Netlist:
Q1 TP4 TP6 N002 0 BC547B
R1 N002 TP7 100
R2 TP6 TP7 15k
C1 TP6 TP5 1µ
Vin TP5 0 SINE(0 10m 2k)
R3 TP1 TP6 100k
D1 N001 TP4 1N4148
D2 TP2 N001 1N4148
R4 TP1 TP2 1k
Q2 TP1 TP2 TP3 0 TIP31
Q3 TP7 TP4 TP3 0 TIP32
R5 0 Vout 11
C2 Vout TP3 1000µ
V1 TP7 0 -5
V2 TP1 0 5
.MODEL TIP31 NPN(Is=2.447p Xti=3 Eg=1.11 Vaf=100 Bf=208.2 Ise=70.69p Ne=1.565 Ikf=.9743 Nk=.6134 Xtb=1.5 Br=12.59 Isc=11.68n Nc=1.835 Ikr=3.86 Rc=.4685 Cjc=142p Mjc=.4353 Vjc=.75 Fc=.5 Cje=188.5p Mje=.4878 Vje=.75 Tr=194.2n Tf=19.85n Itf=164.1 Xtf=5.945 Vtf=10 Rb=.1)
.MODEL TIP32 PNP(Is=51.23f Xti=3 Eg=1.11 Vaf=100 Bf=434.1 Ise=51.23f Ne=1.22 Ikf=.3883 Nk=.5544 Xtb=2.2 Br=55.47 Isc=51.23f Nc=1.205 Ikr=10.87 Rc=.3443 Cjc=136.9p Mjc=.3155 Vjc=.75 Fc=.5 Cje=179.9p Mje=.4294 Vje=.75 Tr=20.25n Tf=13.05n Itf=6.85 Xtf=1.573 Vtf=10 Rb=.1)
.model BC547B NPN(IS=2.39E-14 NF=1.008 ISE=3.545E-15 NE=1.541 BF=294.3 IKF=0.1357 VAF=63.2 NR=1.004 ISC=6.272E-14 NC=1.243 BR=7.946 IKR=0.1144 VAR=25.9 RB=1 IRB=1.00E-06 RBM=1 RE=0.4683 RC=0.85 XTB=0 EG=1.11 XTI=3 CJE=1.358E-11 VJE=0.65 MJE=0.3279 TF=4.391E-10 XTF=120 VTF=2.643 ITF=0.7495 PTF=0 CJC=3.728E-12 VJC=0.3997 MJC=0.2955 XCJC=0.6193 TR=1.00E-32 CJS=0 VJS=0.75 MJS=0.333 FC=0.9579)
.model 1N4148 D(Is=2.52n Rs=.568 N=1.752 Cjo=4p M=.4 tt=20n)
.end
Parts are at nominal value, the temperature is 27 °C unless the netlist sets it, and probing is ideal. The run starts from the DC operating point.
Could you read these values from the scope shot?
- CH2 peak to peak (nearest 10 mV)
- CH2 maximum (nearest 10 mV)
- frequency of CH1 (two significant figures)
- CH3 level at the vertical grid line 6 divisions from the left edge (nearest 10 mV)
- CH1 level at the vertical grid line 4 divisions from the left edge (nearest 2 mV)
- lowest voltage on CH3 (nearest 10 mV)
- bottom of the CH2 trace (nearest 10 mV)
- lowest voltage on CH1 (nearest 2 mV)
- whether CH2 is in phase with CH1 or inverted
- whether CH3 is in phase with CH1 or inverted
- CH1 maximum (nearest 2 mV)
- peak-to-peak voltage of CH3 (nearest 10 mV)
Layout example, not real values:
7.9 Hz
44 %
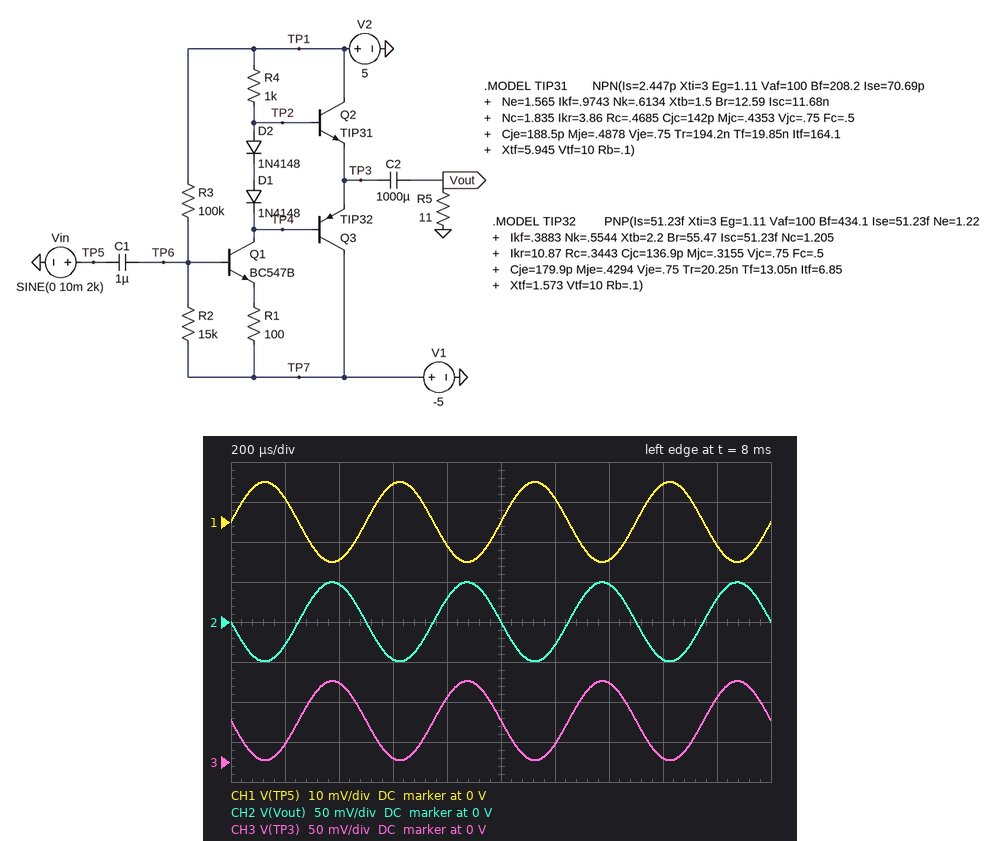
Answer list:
100 mV
50 mV
2.0 kHz
20 mV
-6 mV
0 V
-50 mV
-10 mV
inverted
inverted
10 mV
100 mV
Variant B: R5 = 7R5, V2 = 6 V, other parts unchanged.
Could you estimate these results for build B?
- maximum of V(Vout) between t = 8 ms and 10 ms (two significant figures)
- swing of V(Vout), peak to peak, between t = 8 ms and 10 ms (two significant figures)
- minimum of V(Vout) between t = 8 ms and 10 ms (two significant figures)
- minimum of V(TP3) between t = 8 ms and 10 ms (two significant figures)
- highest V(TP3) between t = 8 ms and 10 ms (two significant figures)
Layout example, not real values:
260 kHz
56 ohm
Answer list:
42 mV
83 mV
-41 mV
150 mV
240 mV
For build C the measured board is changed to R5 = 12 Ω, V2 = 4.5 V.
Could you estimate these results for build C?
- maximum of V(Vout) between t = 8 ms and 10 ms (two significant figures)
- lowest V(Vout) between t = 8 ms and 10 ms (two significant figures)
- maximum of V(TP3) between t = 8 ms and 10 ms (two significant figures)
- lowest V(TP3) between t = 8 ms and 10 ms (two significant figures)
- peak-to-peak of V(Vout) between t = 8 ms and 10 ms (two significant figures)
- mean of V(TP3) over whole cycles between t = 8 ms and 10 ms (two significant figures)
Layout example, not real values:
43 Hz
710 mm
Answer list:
51 mV
-51 mV
32 mV
-70 mV
100 mV
-19 mV
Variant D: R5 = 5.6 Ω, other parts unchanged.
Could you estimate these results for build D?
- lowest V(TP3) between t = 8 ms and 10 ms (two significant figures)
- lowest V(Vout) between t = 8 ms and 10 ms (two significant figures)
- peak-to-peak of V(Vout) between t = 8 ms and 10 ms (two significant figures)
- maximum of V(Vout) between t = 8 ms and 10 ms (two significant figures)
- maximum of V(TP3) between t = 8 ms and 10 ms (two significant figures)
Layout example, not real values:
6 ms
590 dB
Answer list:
18 mV
-34 mV
68 mV
34 mV
86 mV
